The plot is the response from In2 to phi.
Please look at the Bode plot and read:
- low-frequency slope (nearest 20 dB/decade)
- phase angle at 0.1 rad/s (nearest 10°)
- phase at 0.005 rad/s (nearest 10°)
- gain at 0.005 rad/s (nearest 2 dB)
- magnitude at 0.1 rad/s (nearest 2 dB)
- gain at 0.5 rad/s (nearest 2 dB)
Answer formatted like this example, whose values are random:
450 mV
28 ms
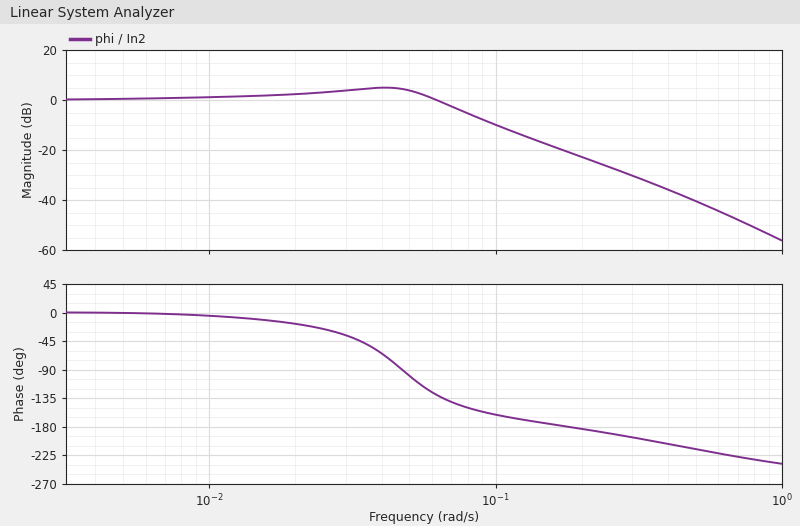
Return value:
0 dB/decade
-160°
0°
0 dB
-10 dB
-40 dB
